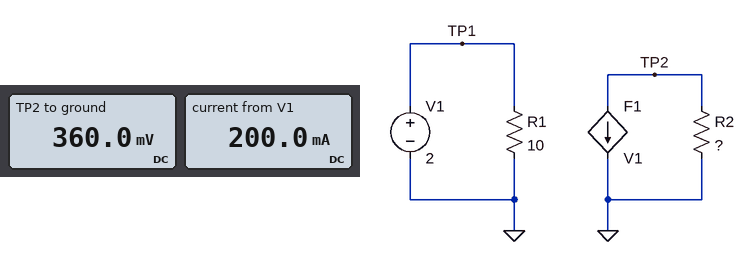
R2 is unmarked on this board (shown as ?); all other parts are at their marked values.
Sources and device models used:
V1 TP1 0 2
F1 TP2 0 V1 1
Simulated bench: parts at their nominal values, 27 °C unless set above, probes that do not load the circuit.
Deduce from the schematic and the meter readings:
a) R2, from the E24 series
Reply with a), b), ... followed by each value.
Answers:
a) 1.8 Ω
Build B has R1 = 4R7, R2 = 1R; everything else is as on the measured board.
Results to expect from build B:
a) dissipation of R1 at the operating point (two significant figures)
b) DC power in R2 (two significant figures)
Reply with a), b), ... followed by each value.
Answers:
a) 850 mW
b) 180 mW
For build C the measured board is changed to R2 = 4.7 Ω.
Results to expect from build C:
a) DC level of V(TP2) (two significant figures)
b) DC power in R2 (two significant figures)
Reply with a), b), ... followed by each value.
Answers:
a) 940 mV
b) 190 mW
